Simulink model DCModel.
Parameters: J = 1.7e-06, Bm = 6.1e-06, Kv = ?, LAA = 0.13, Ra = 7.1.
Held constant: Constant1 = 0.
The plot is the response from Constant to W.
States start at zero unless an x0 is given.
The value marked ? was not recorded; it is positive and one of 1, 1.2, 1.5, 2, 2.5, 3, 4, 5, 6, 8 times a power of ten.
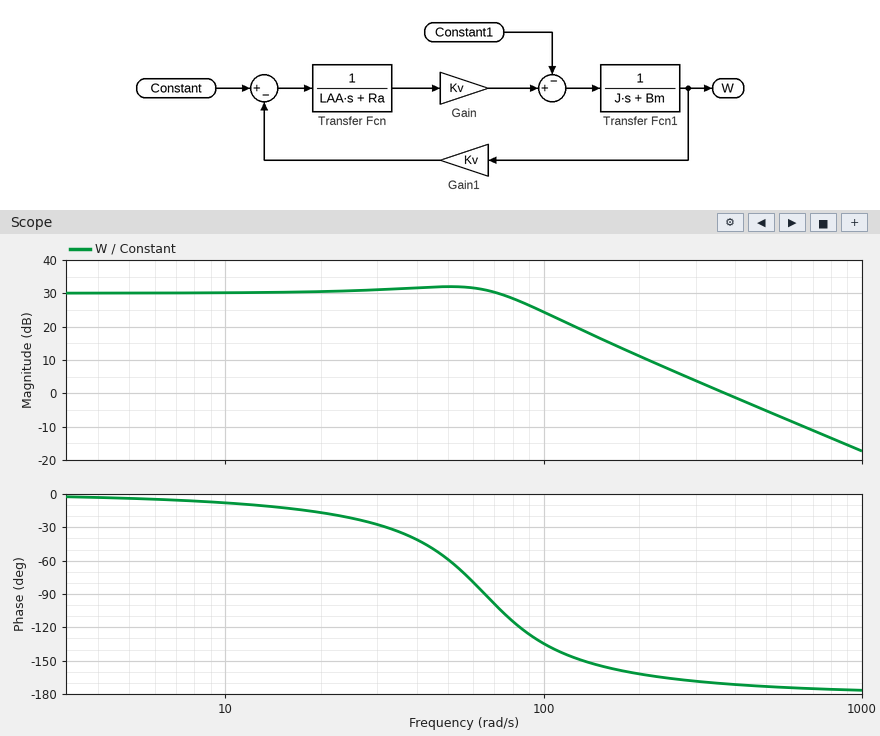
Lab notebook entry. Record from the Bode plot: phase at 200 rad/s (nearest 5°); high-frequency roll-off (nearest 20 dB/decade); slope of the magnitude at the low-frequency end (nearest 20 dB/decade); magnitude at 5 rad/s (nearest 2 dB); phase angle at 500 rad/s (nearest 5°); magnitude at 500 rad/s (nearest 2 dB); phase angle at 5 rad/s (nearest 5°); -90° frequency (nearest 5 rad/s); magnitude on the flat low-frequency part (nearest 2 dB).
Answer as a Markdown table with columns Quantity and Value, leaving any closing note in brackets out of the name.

| Quantity | Value |
|---|---|
| phase at 200 rad/s | -160° |
| high-frequency roll-off | -40 dB/decade |
| slope of the magnitude at the low-frequency end | 0 dB/decade |
| magnitude at 5 rad/s | 30 dB |
| phase angle at 500 rad/s | -175° |
| magnitude at 500 rad/s | -6 dB |
| phase angle at 5 rad/s | -5° |
| -90° frequency | 65 rad/s |
| magnitude on the flat low-frequency part | 30 dB |
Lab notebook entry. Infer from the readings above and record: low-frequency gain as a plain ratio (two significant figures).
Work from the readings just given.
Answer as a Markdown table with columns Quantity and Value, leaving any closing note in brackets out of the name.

| Quantity | Value |
|---|---|
| low-frequency gain as a plain ratio | 32 |
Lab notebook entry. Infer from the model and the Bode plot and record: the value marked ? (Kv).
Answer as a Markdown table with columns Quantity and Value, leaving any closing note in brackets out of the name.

| Quantity | Value |
|---|---|
| the value marked ? | 0.03 |
